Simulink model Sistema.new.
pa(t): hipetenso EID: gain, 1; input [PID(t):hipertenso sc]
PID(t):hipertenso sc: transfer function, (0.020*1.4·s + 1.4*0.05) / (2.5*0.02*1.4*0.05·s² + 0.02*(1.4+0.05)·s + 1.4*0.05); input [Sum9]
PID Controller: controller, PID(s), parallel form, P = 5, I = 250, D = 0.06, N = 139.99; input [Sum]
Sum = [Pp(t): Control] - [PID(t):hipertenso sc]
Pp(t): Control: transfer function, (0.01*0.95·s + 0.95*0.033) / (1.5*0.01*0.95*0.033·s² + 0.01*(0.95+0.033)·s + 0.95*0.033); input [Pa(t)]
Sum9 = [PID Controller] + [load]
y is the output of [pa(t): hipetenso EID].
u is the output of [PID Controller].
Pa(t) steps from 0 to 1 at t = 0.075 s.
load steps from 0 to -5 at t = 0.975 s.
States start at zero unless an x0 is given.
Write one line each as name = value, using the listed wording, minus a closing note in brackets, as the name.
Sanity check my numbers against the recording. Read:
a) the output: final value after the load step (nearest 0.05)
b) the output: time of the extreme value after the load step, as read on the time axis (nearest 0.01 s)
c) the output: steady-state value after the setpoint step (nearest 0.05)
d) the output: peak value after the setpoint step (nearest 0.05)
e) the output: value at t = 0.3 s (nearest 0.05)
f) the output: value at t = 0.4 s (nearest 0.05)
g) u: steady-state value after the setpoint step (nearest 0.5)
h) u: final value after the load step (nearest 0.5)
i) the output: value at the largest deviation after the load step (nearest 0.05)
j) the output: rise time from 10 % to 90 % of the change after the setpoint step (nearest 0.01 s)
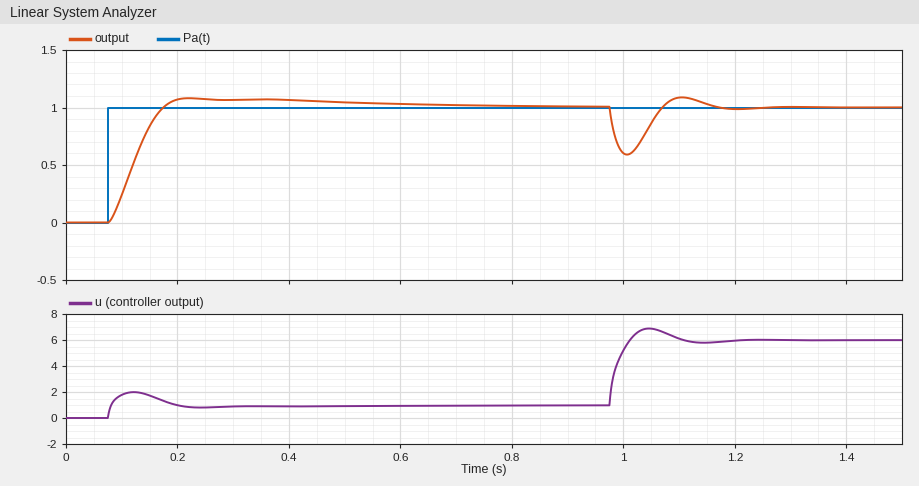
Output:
the output: final value after the load step = 1.00
the output: time of the extreme value after the load step, as read on the time axis = 1.01 s
the output: steady-state value after the setpoint step = 1.00
the output: peak value after the setpoint step = 1.10
the output: value at t = 0.3 s = 1.05
the output: value at t = 0.4 s = 1.05
u: steady-state value after the setpoint step = 1.0
u: final value after the load step = 6.0
the output: value at the largest deviation after the load step = 0.60
the output: rise time from 10 % to 90 % of the change after the setpoint step = 0.07 s
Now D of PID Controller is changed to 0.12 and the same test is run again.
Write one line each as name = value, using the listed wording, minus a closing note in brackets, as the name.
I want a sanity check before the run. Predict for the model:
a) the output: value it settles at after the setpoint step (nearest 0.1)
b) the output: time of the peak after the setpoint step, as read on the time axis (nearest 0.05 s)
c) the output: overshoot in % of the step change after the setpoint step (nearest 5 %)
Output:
the output: value it settles at after the setpoint step = 1.0
the output: time of the peak after the setpoint step, as read on the time axis = 0.25 s
the output: overshoot in % of the step change after the setpoint step = 10 %
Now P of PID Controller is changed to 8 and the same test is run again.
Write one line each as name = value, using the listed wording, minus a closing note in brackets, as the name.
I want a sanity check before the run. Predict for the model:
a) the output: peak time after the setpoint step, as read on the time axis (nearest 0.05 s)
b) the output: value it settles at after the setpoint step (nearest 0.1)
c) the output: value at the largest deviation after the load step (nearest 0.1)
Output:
the output: peak time after the setpoint step, as read on the time axis = 0.25 s
the output: value it settles at after the setpoint step = 1.0
the output: value at the largest deviation after the load step = 0.7
